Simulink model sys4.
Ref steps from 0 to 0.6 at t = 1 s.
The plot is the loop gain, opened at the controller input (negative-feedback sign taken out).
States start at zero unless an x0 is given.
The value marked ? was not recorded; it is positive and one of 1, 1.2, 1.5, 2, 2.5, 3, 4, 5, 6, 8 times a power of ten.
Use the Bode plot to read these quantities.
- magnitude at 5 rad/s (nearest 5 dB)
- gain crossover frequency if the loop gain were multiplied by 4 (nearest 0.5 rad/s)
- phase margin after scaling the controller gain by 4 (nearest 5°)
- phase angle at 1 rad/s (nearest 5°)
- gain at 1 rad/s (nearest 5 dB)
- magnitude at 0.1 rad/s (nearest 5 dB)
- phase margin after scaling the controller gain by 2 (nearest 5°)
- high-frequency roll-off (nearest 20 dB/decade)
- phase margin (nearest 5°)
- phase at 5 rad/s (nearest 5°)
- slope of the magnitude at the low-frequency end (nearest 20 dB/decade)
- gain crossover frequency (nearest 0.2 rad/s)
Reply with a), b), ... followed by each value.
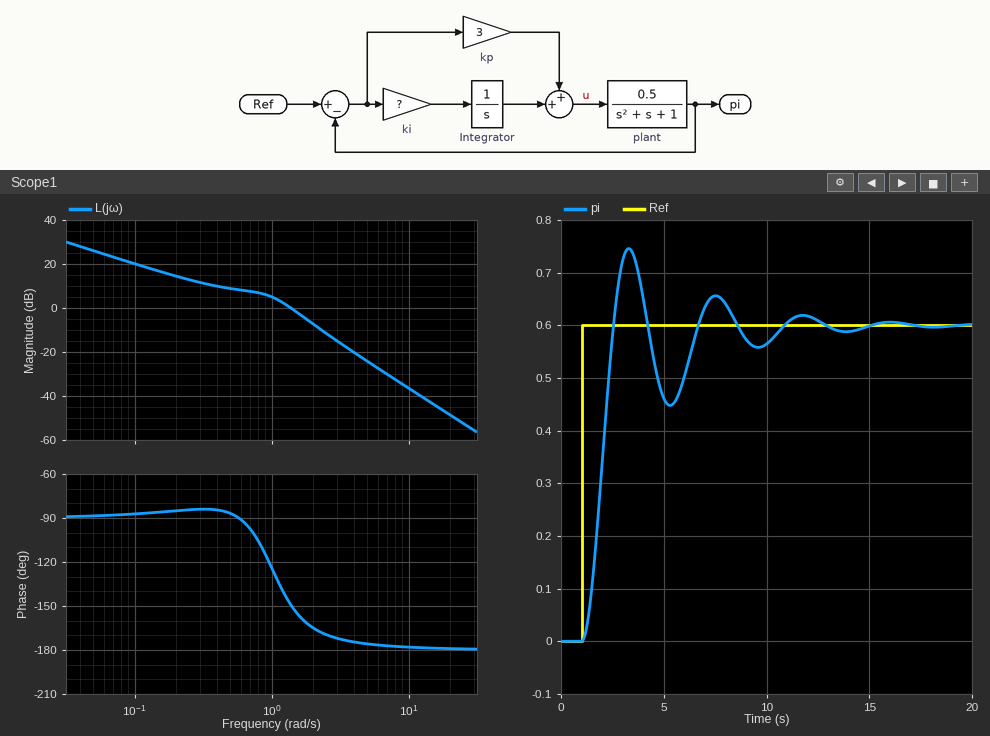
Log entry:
a) -25 dB
b) 2.5 rad/s
c) 10°
d) -125°
e) 5 dB
f) 20 dB
g) 15°
h) -40 dB/decade
i) 30°
j) -175°
k) -20 dB/decade
l) 1.4 rad/s
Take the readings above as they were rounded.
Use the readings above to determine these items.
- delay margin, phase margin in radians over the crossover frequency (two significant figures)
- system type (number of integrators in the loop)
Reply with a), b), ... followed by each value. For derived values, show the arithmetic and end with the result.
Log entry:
a) 30 × π / 180 / 1.4 = 0.37 s
b) 1
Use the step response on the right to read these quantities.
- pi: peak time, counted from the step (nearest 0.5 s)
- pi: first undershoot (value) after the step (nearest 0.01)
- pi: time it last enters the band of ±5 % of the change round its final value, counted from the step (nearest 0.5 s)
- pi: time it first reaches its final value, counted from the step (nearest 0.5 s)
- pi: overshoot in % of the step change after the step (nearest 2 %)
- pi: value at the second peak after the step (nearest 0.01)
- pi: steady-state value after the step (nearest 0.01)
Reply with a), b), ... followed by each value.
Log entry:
a) 2.5 s
b) 0.45
c) 9.0 s
d) 1.5 s
e) 24 %
f) 0.66
g) 0.60
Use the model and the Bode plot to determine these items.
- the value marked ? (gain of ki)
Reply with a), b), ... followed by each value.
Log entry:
a) 2
